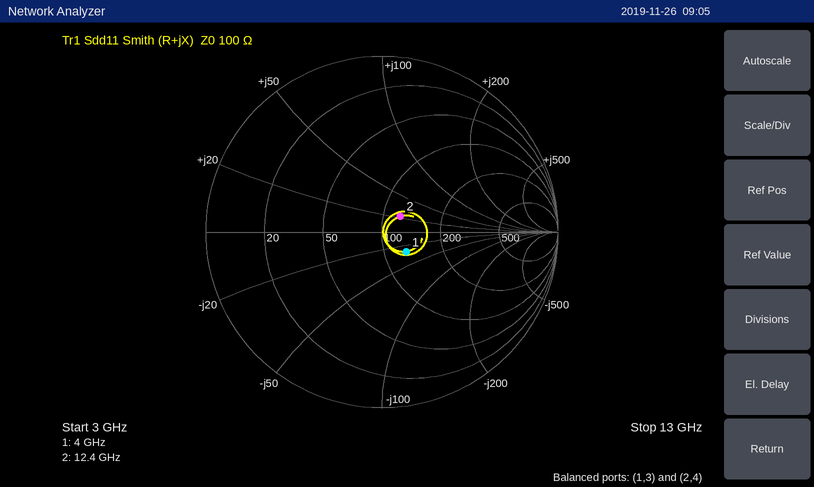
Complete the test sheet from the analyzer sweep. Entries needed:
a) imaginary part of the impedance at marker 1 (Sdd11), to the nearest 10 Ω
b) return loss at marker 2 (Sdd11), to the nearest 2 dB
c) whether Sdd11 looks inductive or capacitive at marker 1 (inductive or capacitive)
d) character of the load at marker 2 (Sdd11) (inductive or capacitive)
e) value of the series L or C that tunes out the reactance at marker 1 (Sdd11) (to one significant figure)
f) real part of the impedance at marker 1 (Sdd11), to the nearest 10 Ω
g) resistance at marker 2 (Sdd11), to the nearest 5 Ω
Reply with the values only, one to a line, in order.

-30 Ω
18 dB
capacitive
inductive
1 nH
130 Ω
120 Ω
